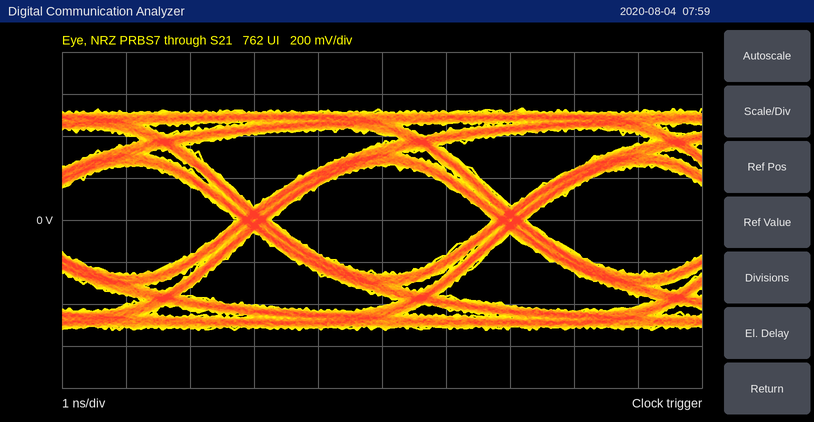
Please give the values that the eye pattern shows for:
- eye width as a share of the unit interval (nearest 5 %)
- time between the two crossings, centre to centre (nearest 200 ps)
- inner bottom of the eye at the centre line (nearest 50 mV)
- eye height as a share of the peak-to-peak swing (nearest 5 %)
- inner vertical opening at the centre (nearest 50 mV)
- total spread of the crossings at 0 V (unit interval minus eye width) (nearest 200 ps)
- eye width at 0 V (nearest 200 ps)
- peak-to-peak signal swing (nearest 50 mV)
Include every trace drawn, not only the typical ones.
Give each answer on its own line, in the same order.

85 %
4.0 ns
-250 mV
50 %
500 mV
600 ps
3.4 ns
1.05 V
